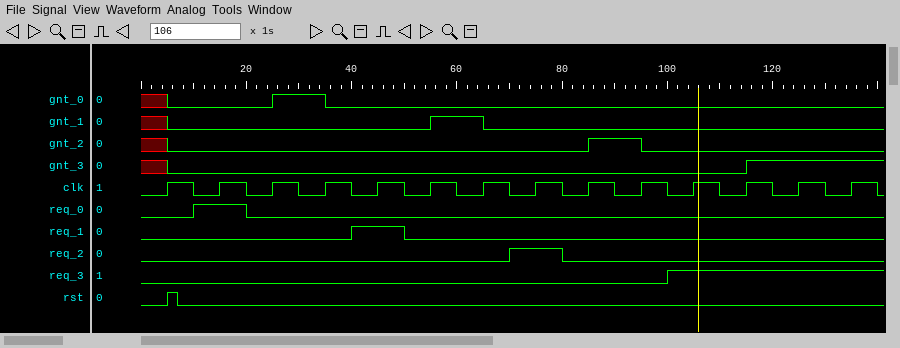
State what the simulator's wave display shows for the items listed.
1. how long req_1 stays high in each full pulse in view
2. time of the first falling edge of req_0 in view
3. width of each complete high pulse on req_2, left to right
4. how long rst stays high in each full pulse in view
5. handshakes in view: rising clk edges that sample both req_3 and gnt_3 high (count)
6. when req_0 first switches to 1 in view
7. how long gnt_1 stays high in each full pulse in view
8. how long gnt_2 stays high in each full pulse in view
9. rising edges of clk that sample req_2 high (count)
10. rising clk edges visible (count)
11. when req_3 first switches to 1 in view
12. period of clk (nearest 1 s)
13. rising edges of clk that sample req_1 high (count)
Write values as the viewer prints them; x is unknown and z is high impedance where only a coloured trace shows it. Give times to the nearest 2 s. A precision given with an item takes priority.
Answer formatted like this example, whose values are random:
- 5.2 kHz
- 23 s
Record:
- 10 s
- 20 s
- 10 s
- 2 s
- 2
- 10 s
- 10 s
- 10 s
- 1
- 14
- 100 s
- 10 s
- 1
